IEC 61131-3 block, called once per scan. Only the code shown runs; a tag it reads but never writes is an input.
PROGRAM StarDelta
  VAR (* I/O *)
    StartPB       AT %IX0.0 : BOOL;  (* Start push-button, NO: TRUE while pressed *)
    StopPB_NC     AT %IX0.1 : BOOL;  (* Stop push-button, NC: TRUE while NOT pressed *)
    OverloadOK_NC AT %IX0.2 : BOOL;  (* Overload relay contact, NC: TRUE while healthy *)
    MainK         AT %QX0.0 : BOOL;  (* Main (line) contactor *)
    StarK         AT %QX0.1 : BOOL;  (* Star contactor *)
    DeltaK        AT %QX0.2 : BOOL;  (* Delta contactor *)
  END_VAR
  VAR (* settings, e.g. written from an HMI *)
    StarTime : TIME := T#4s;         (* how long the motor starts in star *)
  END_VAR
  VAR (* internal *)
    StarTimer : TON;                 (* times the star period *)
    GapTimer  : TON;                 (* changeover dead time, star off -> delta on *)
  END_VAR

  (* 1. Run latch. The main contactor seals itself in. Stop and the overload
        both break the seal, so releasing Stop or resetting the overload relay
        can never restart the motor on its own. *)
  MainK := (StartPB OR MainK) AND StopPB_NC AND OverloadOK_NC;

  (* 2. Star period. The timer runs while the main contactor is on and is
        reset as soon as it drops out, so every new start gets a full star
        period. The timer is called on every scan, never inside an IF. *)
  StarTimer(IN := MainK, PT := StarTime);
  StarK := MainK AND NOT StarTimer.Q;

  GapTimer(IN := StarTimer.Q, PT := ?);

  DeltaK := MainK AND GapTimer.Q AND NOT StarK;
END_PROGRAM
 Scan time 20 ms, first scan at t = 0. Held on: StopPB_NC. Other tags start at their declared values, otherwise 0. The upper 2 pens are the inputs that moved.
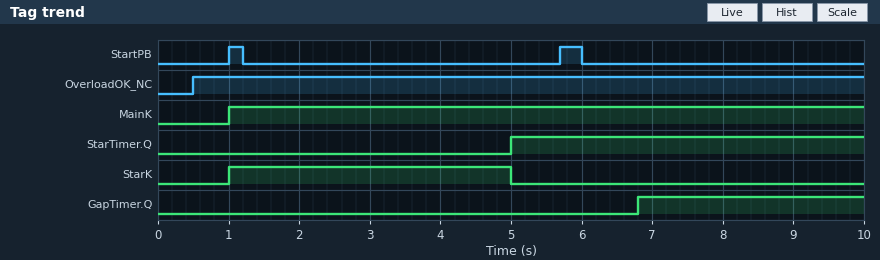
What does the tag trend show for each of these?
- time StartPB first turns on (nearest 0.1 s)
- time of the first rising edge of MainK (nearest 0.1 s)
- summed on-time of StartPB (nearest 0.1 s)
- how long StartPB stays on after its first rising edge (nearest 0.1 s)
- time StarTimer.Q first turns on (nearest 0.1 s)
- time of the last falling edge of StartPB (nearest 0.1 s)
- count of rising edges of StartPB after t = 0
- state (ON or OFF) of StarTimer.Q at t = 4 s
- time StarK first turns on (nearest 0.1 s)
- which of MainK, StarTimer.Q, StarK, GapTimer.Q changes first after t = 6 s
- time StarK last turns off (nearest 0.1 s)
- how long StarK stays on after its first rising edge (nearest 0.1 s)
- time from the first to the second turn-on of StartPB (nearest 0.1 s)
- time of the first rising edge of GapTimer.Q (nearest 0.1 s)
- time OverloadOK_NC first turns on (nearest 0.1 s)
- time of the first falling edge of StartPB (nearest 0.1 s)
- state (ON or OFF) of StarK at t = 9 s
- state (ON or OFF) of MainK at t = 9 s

1.0 s
1.0 s
0.5 s
0.2 s
5.0 s
6.0 s
2
OFF
1.0 s
GapTimer.Q
5.0 s
4.0 s
4.7 s
6.8 s
0.5 s
1.2 s
OFF
ON
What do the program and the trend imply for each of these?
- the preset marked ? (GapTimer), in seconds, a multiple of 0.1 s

1.8 s
